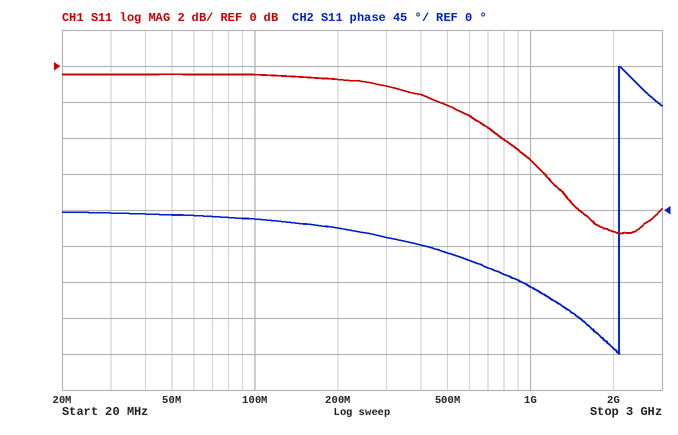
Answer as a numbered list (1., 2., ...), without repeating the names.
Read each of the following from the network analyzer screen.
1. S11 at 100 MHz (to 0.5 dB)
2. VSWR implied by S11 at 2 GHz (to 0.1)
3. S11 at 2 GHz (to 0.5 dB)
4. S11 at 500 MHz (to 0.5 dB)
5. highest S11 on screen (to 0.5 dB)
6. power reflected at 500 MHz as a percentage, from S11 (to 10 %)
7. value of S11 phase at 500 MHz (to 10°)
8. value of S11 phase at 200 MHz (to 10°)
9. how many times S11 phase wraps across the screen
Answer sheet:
1. -0.5 dB
2. 2.1
3. -9.0 dB
4. -2.0 dB
5. -0.5 dB
6. 60 %
7. -50°
8. -20°
9. 1
